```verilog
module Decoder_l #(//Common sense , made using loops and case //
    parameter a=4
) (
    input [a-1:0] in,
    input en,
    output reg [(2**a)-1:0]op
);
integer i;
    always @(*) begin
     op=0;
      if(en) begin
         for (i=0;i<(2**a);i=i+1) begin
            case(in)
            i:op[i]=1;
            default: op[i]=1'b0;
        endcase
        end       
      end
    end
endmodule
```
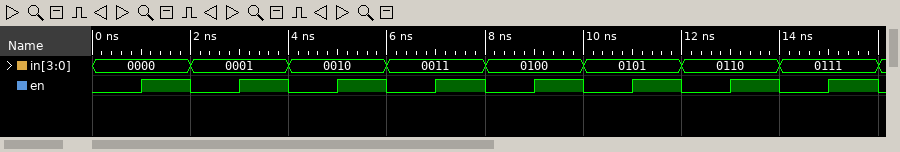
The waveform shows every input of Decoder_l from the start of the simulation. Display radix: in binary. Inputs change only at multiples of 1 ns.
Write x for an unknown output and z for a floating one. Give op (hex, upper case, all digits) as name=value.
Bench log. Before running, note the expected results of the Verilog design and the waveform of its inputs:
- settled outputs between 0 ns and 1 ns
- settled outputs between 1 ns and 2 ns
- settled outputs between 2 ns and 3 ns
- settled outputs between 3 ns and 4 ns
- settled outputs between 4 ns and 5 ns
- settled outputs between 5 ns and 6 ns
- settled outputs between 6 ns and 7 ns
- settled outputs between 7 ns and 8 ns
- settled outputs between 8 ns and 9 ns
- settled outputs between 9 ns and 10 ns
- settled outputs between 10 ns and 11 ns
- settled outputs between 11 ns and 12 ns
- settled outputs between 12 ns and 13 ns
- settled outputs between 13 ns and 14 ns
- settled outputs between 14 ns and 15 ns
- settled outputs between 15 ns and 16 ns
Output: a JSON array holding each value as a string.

["op=0000", "op=0001", "op=0000", "op=0002", "op=0000", "op=0004", "op=0000", "op=0008", "op=0000", "op=0010", "op=0000", "op=0020", "op=0000", "op=0040", "op=0000", "op=0080"]
